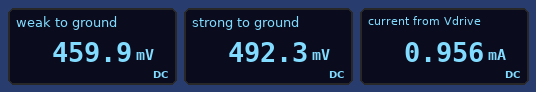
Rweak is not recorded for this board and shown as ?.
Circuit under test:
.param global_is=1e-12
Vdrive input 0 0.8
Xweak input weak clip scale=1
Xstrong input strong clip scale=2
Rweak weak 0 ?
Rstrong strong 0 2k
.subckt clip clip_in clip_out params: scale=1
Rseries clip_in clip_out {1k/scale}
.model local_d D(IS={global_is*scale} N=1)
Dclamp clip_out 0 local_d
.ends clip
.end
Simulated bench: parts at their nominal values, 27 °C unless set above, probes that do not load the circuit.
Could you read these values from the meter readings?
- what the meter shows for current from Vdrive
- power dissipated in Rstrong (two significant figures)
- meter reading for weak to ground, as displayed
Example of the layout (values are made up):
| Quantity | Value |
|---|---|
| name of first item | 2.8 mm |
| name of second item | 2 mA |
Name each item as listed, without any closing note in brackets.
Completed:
| Quantity | Value |
|---|---|
| what the meter shows for current from Vdrive | 0.956 mA |
| power dissipated in Rstrong | 120 µW |
| meter reading for weak to ground, as displayed | 459.9 mV |
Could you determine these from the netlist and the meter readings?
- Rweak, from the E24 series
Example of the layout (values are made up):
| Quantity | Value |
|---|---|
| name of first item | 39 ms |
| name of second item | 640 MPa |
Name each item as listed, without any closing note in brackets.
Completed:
| Quantity | Value |
|---|---|
| Rweak, from the E24 series | 1.6 kΩ |
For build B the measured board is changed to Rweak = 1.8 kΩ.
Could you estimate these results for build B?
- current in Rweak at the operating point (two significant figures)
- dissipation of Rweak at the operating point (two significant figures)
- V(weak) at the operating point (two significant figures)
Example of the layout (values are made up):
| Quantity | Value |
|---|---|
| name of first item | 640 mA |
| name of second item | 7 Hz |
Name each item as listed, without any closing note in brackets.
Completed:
| Quantity | Value |
|---|---|
| current in Rweak at the operating point | 260 µA |
| dissipation of Rweak at the operating point | 120 µW |
| V(weak) at the operating point | 470 mV |
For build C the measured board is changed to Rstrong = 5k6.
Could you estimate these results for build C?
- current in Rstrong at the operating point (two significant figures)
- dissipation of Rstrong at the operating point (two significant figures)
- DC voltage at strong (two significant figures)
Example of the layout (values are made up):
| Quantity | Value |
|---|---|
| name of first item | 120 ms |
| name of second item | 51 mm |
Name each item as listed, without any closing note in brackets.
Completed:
| Quantity | Value |
|---|---|
| current in Rstrong at the operating point | 89 µA |
| dissipation of Rstrong at the operating point | 45 µW |
| DC voltage at strong | 500 mV |
